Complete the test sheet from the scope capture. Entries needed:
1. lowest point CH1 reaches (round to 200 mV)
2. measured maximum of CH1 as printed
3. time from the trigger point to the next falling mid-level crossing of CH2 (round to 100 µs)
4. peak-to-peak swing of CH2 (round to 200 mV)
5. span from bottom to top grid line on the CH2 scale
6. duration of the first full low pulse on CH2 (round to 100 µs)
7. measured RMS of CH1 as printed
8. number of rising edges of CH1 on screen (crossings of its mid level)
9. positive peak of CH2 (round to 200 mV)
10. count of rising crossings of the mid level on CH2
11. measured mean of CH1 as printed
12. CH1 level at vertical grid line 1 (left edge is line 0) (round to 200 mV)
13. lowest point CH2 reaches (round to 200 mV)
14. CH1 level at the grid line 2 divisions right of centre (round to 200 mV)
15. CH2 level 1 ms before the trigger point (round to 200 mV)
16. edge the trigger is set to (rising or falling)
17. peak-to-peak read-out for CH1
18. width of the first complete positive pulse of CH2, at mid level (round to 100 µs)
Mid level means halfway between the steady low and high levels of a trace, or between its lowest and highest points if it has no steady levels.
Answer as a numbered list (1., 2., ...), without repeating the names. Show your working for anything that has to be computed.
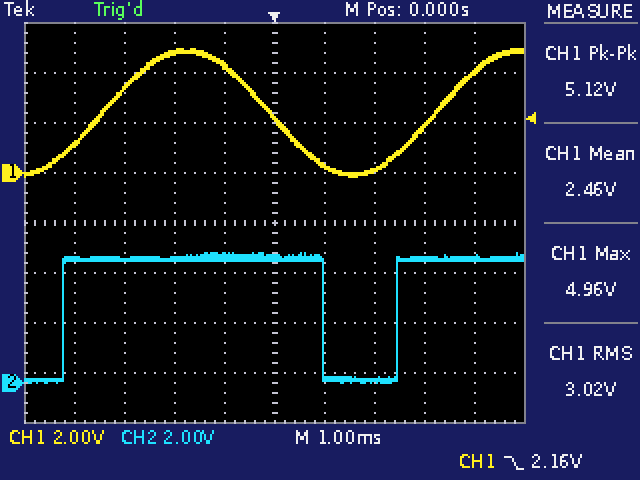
1. -200 mV
2. 4.96 V
3. 1.0 ms
4. 5.2 V − (0.0 V) = 5.2 V
5. 16 V
6. 1.5 ms
7. 3.02 V
8. 2
9. 5.2 V
10. 2
11. 2.46 V
12. 1.2 V
13. 0.0 V
14. 200 mV
15. 5.0 V
16. falling
17. 5.12 V
18. 5.2 ms
